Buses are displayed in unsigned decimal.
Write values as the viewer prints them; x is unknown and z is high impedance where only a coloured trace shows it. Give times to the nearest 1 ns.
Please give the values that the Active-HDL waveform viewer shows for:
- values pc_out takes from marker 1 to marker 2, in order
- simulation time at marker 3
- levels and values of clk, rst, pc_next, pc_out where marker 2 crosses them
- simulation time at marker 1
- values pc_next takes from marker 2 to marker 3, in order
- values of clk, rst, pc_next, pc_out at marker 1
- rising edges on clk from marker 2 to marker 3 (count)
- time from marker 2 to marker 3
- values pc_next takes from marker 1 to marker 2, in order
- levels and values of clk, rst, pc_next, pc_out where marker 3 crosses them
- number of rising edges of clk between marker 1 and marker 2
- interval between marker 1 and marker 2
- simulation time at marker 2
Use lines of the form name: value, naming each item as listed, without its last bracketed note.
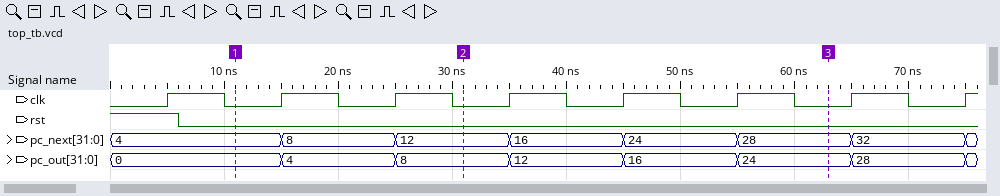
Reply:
values pc_out takes from marker 1 to marker 2, in order: 0, 4, 8
simulation time at marker 3: 63 ns
levels and values of clk, rst, pc_next, pc_out where marker 2 crosses them: clk=0, rst=0, pc_next=12, pc_out=8
simulation time at marker 1: 11 ns
values pc_next takes from marker 2 to marker 3, in order: 12, 16, 24, 28
values of clk, rst, pc_next, pc_out at marker 1: clk=0, rst=0, pc_next=4, pc_out=0
rising edges on clk from marker 2 to marker 3: 3
time from marker 2 to marker 3: 32 ns
values pc_next takes from marker 1 to marker 2, in order: 4, 8, 12
levels and values of clk, rst, pc_next, pc_out where marker 3 crosses them: clk=0, rst=0, pc_next=28, pc_out=24
number of rising edges of clk between marker 1 and marker 2: 2
interval between marker 1 and marker 2: 20 ns
simulation time at marker 2: 31 ns
